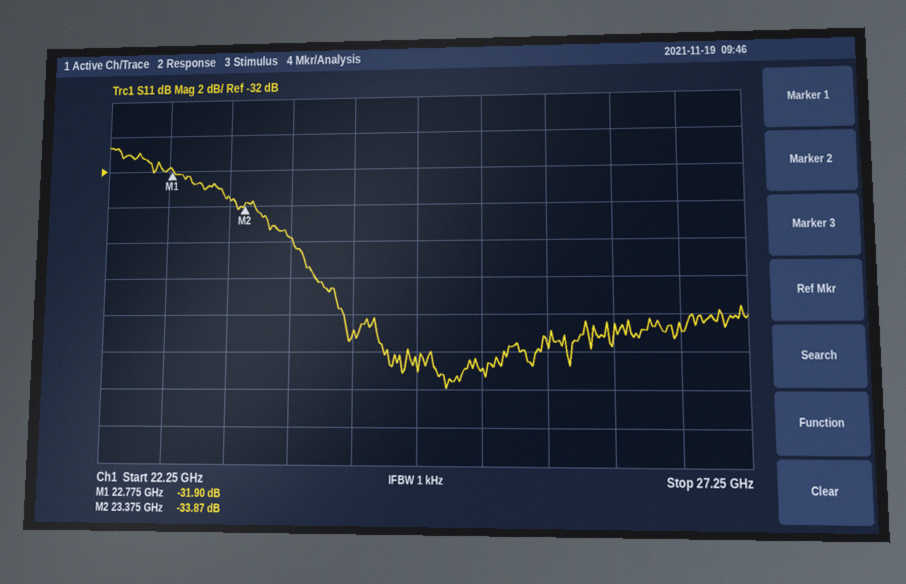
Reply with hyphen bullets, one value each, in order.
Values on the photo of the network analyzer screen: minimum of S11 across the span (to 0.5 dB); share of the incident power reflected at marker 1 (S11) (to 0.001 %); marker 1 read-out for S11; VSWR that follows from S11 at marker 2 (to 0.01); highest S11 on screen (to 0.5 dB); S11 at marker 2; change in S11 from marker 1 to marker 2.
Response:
- -44.0 dB
- 0.065 %
- -31.90 dB
- 1.04
- -30.5 dB
- -33.87 dB
- -1.97 dB
